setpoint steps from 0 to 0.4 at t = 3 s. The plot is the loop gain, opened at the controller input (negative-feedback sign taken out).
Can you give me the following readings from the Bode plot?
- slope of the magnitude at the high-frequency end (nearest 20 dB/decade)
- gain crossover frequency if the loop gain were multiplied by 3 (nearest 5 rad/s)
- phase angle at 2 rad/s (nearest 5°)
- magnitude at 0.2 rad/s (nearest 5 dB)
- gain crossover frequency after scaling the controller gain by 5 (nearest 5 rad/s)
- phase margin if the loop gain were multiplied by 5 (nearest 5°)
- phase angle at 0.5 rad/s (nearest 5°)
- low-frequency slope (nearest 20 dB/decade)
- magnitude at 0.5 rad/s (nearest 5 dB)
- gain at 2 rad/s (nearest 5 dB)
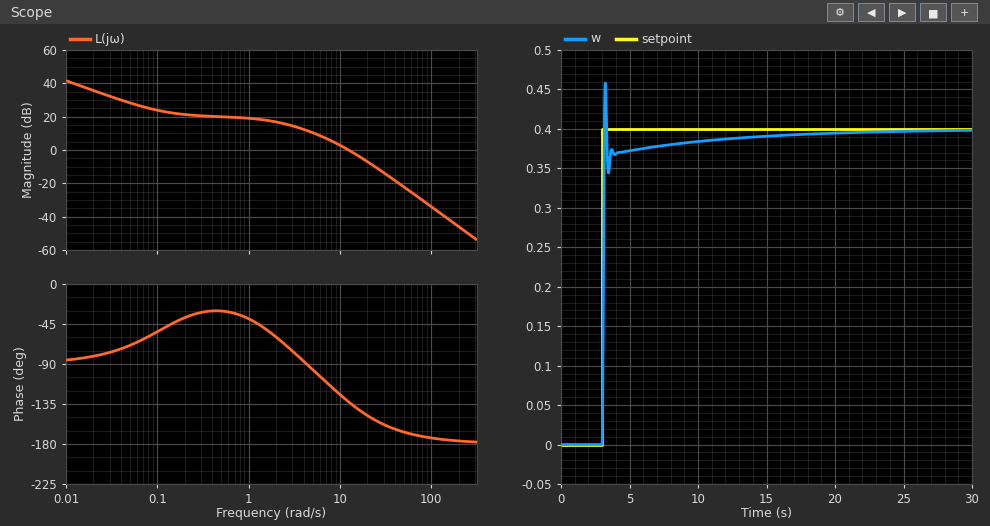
-40 dB/decade
25 rad/s
-60°
20 dB
30 rad/s
20°
-30°
-20 dB/decade
20 dB
15 dB
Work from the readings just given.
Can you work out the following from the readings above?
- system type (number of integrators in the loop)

1
